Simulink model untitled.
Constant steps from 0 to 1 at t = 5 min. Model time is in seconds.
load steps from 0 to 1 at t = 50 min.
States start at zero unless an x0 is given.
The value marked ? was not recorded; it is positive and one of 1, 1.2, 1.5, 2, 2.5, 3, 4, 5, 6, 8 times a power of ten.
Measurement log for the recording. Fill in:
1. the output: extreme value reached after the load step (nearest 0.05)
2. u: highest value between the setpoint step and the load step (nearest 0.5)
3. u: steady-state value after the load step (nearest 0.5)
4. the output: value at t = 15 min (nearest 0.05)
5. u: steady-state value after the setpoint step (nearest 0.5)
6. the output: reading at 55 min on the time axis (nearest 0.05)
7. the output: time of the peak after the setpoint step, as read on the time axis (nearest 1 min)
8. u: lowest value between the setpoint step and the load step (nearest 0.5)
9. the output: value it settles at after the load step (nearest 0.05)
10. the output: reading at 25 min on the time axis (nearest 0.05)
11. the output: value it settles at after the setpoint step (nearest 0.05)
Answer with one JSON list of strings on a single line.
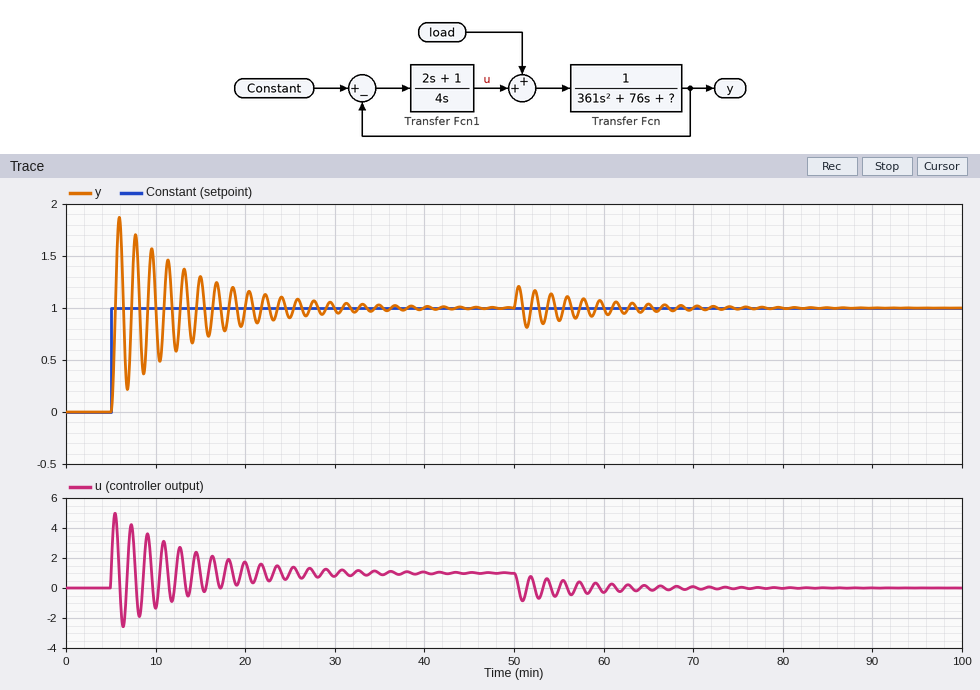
["1.20", "5.0", "0.0", "1.30", "1.0", "0.90", "6 min", "-2.5", "1.00", "0.90", "1.00"]
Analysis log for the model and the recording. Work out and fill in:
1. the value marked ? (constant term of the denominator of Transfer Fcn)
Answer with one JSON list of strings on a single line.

["1"]
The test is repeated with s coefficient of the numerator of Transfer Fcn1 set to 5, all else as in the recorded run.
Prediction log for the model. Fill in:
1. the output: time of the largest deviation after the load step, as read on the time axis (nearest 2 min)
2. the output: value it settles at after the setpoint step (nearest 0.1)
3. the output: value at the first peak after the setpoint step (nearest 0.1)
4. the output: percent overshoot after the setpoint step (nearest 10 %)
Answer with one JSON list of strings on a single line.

["50 min", "1.0", "1.7", "70 %"]
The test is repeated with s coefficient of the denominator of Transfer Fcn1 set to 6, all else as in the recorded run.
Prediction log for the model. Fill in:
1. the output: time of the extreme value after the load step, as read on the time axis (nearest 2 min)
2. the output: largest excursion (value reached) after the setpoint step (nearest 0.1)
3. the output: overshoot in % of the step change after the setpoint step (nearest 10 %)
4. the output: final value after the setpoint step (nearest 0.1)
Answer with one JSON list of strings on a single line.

["50 min", "1.8", "80 %", "1.0"]
